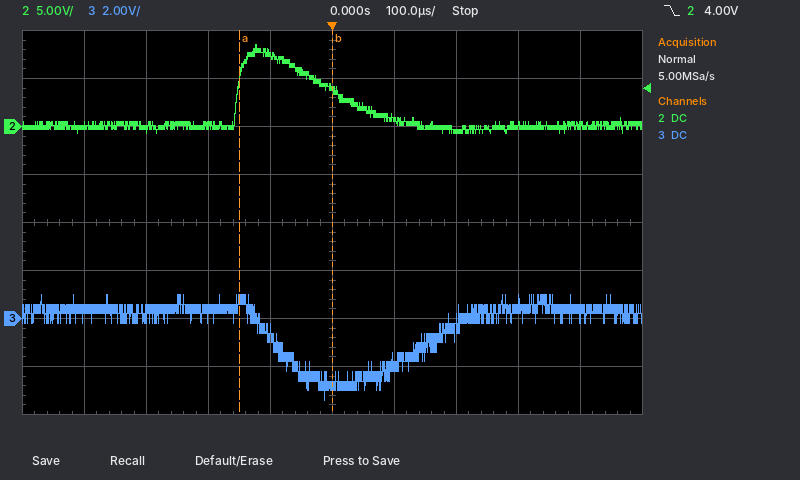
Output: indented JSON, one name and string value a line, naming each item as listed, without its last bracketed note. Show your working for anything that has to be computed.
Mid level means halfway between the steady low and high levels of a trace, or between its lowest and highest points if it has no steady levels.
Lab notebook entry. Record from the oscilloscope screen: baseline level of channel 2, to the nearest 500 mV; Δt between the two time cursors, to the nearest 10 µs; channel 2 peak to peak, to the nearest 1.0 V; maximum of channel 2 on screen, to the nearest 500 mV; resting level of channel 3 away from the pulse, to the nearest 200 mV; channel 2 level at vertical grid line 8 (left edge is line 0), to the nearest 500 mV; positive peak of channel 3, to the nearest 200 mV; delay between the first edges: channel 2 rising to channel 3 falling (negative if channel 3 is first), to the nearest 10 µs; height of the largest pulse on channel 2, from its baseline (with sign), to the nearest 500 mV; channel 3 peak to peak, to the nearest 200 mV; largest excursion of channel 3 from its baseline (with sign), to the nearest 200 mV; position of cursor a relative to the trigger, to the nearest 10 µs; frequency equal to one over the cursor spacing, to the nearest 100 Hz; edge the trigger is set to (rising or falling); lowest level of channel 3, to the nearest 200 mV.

{
  "baseline level of channel 2, to the nearest 500 mV": "0.0 V",
  "Δt between the two time cursors, to the nearest 10 µs": "150 µs",
  "channel 2 peak to peak, to the nearest 1.0 V": "9.0 V",
  "maximum of channel 2 on screen, to the nearest 500 mV": "8.5 V",
  "resting level of channel 3 away from the pulse, to the nearest 200 mV": "400 mV",
  "channel 2 level at vertical grid line 8 (left edge is line 0), to the nearest 500 mV": "0.0 V",
  "positive peak of channel 3, to the nearest 200 mV": "1.0 V",
  "delay between the first edges: channel 2 rising to channel 3 falling (negative if channel 3 is first), to the nearest 10 µs": "+60 µs",
  "height of the largest pulse on channel 2, from its baseline (with sign), to the nearest 500 mV": "8.5 V − (0.0 V) = +8.5 V",
  "channel 3 peak to peak, to the nearest 200 mV": "1.0 V − (-3.4 V) = 4.4 V",
  "largest excursion of channel 3 from its baseline (with sign), to the nearest 200 mV": "-3.4 V − (400 mV) = -3.8 V",
  "position of cursor a relative to the trigger, to the nearest 10 µs": "-150 µs",
  "frequency equal to one over the cursor spacing, to the nearest 100 Hz": "1 / 150 µs ≈ 6.7 kHz",
  "edge the trigger is set to": "falling",
  "lowest level of channel 3, to the nearest 200 mV": "-3.4 V"
}
